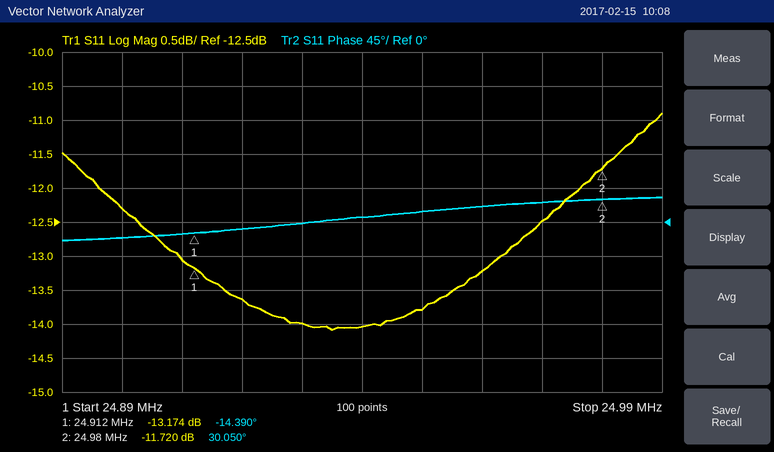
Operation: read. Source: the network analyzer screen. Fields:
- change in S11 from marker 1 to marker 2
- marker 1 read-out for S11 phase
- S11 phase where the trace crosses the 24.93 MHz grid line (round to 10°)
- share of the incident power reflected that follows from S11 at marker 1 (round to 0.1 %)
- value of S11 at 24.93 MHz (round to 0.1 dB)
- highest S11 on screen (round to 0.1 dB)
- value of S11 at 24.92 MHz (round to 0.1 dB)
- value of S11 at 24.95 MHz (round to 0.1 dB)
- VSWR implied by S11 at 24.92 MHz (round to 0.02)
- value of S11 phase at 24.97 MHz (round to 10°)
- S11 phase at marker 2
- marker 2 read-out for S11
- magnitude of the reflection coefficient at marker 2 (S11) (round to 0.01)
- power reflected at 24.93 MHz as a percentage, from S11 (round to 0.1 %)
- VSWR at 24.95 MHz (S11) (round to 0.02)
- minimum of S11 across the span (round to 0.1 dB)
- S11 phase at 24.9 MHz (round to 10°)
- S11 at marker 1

1.454 dB
-14.390°
0°
4.8 %
-14.0 dB
-10.9 dB
-13.6 dB
-13.8 dB
1.52
30°
30.050°
-11.720 dB
0.26
4.0 %
1.52
-14.1 dB
-20°
-13.174 dB
